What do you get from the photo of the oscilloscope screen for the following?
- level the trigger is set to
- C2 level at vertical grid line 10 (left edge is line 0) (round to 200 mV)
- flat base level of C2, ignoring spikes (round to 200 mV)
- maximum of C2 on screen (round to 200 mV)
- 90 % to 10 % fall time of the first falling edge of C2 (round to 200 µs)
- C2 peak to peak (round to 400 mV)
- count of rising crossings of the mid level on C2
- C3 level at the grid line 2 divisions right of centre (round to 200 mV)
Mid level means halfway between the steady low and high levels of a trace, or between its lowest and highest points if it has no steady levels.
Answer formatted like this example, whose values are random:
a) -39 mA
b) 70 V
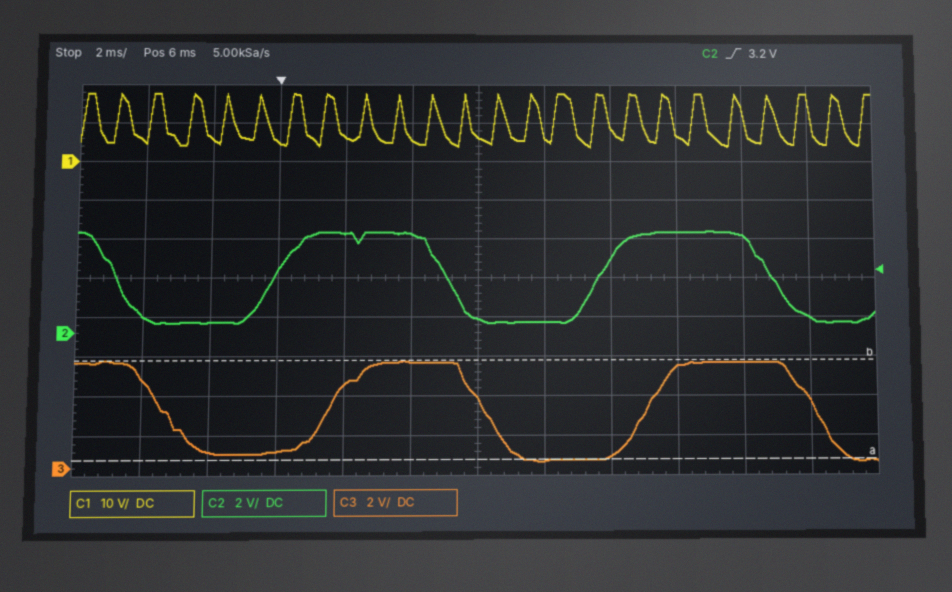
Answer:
a) 3.2 V
b) 5.0 V
c) 600 mV
d) 5.2 V
e) 1.4 ms
f) 4.8 V
g) 2
h) 600 mV
